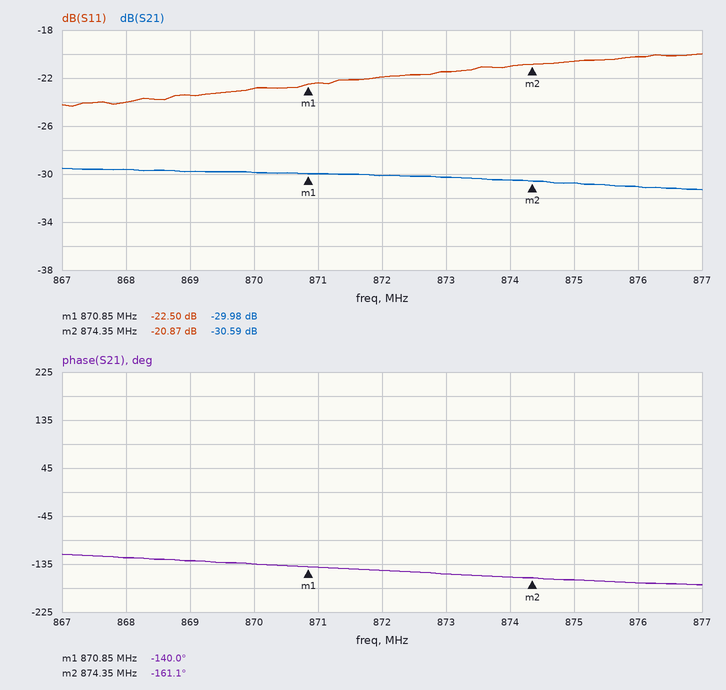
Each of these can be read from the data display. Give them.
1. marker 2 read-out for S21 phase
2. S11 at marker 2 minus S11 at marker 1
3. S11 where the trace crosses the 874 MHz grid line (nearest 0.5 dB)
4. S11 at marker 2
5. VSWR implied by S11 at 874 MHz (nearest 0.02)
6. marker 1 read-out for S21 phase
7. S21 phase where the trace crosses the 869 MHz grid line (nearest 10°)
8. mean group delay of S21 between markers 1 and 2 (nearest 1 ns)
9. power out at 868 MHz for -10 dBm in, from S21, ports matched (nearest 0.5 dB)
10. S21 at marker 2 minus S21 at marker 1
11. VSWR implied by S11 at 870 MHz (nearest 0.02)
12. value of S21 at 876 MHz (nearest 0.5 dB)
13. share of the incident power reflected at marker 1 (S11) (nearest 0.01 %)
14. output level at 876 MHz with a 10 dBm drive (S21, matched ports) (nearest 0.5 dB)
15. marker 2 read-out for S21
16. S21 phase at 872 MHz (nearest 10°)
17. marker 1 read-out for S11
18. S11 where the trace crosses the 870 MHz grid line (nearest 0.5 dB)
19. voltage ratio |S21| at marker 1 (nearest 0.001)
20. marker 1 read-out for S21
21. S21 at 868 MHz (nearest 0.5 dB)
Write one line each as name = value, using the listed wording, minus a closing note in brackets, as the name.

marker 2 read-out for S21 phase = -161.1°
S11 at marker 2 minus S11 at marker 1 = 1.63 dB
S11 where the trace crosses the 874 MHz grid line = -21.0 dB
S11 at marker 2 = -20.87 dB
VSWR implied by S11 at 874 MHz = 1.20
marker 1 read-out for S21 phase = -140.0°
S21 phase where the trace crosses the 869 MHz grid line = -130°
mean group delay of S21 between markers 1 and 2 = 17 ns
power out at 868 MHz for -10 dBm in, from S21, ports matched = -39.5 dBm
S21 at marker 2 minus S21 at marker 1 = -0.61 dB
VSWR implied by S11 at 870 MHz = 1.16
value of S21 at 876 MHz = -31.0 dB
share of the incident power reflected at marker 1 (S11) = 0.56 %
output level at 876 MHz with a 10 dBm drive (S21, matched ports) = -21.0 dBm
marker 2 read-out for S21 = -30.59 dB
S21 phase at 872 MHz = -150°
marker 1 read-out for S11 = -22.50 dB
S11 where the trace crosses the 870 MHz grid line = -23.0 dB
voltage ratio |S21| at marker 1 = 0.032
marker 1 read-out for S21 = -29.98 dB
S21 at 868 MHz = -29.5 dB
